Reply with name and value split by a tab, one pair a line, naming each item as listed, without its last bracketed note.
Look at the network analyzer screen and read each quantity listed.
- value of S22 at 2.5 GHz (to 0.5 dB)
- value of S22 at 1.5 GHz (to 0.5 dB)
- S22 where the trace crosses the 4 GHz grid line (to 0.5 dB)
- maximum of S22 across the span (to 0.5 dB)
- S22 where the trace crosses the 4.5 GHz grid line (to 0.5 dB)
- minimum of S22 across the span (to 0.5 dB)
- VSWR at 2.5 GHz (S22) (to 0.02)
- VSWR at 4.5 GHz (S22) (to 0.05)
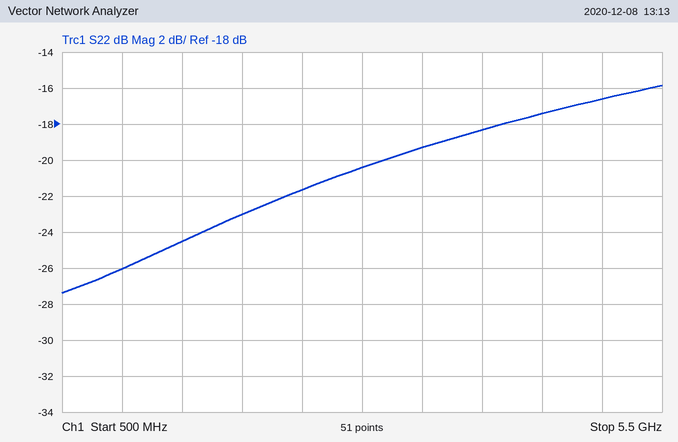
value of S22 at 2.5 GHz	-21.5 dB
value of S22 at 1.5 GHz	-24.5 dB
S22 where the trace crosses the 4 GHz grid line	-18.5 dB
maximum of S22 across the span	-16.0 dB
S22 where the trace crosses the 4.5 GHz grid line	-17.5 dB
minimum of S22 across the span	-27.5 dB
VSWR at 2.5 GHz (S22)	1.18
VSWR at 4.5 GHz (S22)	1.30
